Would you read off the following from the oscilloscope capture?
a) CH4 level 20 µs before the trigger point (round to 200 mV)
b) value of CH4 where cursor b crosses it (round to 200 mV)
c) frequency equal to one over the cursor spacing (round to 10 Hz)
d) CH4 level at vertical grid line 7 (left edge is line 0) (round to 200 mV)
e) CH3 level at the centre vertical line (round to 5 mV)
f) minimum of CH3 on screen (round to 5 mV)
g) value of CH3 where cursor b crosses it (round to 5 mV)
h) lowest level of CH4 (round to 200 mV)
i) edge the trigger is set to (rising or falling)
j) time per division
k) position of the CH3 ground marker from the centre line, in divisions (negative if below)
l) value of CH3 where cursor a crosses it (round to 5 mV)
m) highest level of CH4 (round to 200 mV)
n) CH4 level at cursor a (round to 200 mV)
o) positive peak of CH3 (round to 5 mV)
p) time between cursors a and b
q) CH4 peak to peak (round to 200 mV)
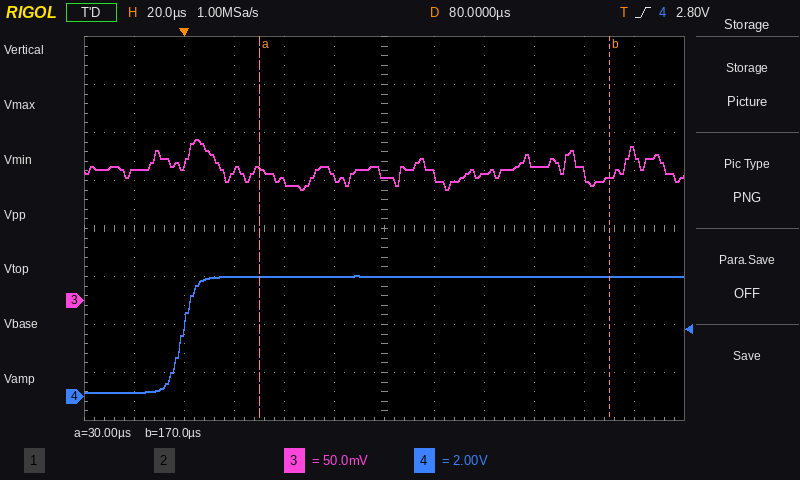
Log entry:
200 mV
5.0 V
7.14 kHz
5.0 V
130 mV
115 mV
130 mV
200 mV
rising
20 µs
-1.5 div
140 mV
5.0 V
5.0 V
170 mV
140 µs
4.8 V
